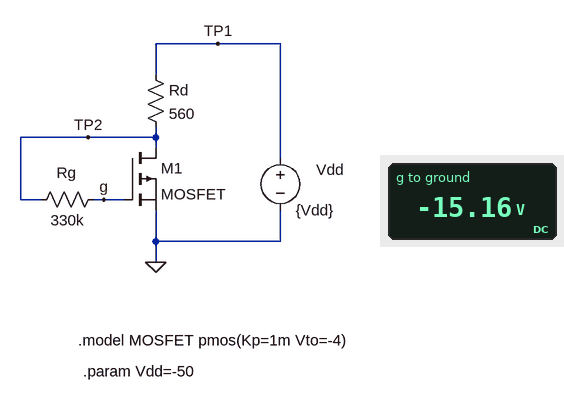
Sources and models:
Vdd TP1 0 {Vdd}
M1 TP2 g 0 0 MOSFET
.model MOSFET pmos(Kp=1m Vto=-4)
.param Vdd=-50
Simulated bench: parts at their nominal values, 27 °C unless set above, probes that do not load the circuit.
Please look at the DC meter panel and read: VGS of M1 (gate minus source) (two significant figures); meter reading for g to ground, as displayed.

-15 V
-15.16 V
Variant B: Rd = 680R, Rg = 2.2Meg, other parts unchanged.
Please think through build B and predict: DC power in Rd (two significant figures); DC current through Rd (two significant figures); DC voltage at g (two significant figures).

1.9 W
53 mA
-14 V
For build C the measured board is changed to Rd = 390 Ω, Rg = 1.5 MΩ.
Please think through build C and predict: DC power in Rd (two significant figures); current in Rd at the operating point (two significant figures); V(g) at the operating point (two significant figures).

2.8 W
85 mA
-17 V
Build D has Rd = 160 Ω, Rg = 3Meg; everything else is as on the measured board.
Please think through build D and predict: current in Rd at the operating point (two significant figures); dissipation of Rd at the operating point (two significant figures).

170 mA
4.7 W
